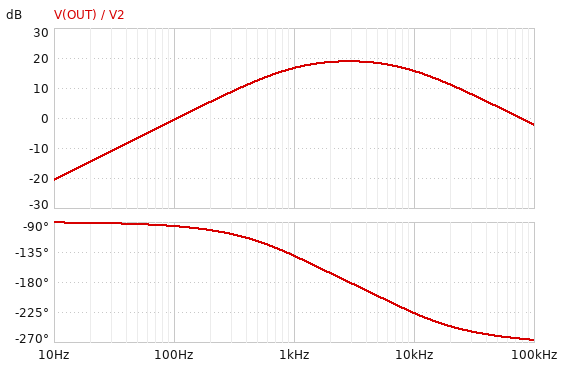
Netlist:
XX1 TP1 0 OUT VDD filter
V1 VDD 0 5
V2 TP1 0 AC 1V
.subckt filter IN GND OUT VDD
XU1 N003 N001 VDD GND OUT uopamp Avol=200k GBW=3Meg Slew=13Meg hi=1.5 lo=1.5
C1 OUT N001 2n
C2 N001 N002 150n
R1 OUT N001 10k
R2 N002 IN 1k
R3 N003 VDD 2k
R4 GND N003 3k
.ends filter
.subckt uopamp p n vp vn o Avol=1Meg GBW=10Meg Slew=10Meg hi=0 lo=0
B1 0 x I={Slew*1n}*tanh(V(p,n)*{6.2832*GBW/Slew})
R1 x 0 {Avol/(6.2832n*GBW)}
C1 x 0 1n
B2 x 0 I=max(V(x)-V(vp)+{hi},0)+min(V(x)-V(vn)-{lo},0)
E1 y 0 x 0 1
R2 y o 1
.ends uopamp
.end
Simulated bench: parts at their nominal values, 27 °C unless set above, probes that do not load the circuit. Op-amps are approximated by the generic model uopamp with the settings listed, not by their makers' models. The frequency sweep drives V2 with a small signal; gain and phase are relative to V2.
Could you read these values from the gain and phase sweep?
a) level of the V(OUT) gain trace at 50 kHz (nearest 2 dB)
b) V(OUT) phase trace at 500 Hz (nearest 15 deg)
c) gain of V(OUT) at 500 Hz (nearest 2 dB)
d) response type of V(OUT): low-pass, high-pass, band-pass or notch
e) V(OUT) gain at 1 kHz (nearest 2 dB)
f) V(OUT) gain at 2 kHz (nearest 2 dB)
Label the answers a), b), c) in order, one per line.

a) 4 dB
b) -120 deg
c) 12 dB
d) band-pass
e) 16 dB
f) 18 dB
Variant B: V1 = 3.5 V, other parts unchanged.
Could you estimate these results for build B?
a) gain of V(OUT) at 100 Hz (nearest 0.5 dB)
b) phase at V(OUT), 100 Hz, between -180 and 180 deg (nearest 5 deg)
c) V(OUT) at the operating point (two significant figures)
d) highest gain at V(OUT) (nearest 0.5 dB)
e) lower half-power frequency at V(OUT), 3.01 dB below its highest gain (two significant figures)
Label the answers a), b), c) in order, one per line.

a) -38.5 dB
b) -135 deg
c) 2.0 V
d) -35.5 dB
e) 97 Hz
